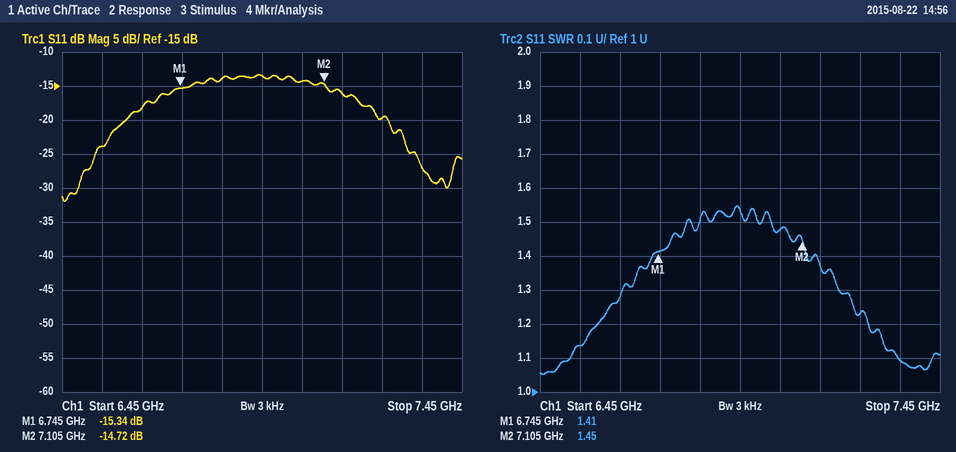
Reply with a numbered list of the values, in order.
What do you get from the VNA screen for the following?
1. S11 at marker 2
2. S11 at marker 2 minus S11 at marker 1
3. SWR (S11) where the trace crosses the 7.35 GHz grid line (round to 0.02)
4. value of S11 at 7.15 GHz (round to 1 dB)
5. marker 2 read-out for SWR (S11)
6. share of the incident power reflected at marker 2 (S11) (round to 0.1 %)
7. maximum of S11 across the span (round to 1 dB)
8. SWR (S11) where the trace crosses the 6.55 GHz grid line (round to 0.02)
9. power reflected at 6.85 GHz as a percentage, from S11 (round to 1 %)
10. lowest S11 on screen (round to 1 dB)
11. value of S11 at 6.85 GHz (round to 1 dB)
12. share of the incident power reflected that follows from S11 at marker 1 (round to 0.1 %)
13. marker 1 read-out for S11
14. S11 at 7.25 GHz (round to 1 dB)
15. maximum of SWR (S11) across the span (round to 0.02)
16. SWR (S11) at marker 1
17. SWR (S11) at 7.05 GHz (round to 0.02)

1. -14.72 dB
2. 0.62 dB
3. 1.10
4. -16 dB
5. 1.45
6. 3.4 %
7. -13 dB
8. 1.14
9. 4 %
10. -32 dB
11. -14 dB
12. 2.9 %
13. -15.34 dB
14. -20 dB
15. 1.54
16. 1.41
17. 1.48
